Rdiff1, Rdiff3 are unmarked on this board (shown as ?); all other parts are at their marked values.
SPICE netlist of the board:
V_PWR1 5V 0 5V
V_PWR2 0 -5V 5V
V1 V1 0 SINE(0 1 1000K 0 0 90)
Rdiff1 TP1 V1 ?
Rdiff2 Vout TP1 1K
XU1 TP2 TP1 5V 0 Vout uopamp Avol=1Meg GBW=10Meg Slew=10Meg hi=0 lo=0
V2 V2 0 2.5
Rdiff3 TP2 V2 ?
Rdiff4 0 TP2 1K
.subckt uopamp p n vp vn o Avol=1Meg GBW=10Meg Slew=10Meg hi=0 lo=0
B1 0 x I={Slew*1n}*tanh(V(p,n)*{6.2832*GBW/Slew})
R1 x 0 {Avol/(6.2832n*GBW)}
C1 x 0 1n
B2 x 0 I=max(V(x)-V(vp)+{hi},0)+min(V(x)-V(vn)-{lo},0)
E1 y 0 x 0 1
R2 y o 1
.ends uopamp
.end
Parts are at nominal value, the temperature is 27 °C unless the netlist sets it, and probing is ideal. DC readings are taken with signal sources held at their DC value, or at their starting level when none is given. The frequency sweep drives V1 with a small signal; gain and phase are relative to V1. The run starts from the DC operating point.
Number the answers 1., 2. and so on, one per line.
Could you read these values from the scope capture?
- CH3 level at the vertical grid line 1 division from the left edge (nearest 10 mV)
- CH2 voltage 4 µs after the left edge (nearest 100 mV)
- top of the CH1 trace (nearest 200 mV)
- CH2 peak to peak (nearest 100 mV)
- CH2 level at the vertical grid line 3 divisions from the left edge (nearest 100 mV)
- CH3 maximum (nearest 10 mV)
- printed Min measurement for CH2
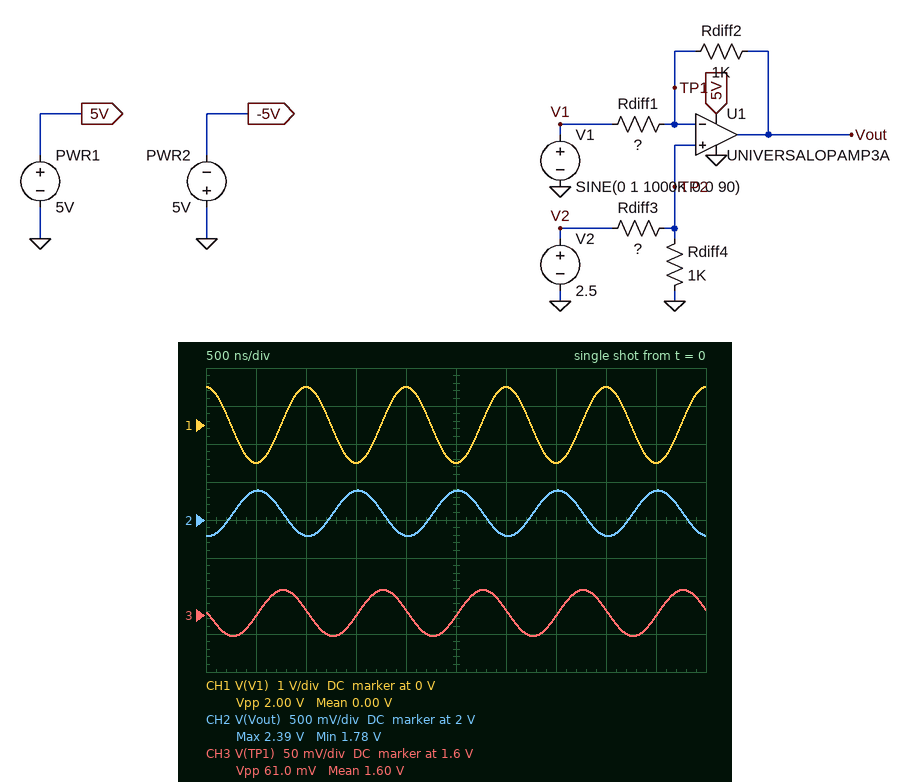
1. 1.60 V
2. 1.8 V
3. 1.0 V
4. 600 mV
5. 2.4 V
6. 1.63 V
7. 1.78 V
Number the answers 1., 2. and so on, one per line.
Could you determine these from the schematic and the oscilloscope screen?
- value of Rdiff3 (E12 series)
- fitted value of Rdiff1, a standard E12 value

1. 560 Ω
2. 3.3 kΩ
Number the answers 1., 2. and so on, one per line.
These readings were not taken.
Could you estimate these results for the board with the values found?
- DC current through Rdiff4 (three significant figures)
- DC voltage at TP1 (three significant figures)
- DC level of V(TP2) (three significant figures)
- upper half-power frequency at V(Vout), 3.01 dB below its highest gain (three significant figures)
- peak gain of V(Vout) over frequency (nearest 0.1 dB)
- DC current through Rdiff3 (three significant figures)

1. 1.60 mA
2. 1.60 V
3. 1.60 V
4. 7.67 MHz
5. -10.4 dB
6. 1.60 mA
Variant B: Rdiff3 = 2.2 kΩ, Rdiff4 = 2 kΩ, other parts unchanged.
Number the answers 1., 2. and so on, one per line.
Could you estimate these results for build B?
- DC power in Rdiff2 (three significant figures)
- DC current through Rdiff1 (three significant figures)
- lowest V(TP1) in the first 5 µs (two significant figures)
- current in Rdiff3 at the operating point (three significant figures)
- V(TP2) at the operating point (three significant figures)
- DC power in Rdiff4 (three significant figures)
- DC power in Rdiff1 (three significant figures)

1. 3.33 µW
2. 57.7 µA
3. 1.2 V
4. 595 µA
5. 1.19 V
6. 709 µW
7. 11.0 µW
